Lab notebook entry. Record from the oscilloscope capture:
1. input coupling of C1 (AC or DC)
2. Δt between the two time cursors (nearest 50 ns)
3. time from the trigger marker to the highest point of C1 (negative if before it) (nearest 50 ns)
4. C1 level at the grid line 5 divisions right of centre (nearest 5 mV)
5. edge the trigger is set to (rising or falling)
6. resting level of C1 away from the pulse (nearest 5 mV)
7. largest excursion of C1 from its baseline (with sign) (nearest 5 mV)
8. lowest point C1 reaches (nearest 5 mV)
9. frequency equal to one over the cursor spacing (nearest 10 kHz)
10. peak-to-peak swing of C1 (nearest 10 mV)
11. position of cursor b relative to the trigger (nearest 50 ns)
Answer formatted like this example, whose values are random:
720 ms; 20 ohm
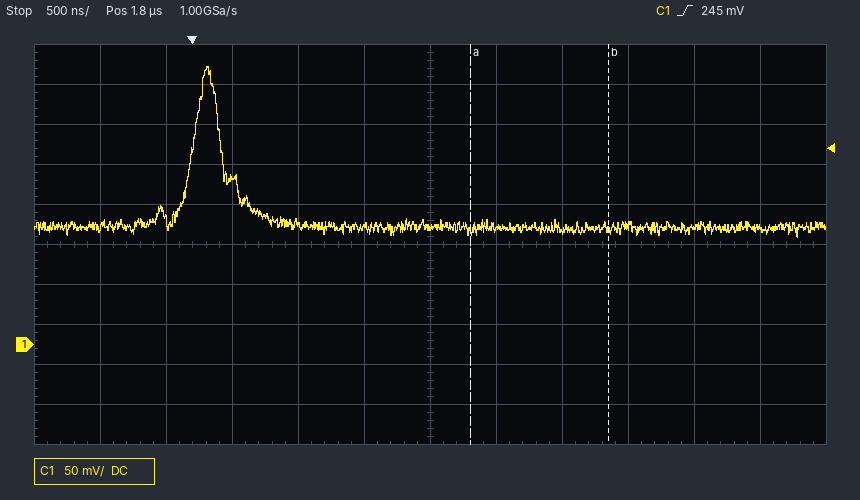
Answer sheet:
DC; 1.05 µs; +100 ns; 145 mV; rising; 145 mV; +200 mV; 135 mV; 950 kHz; 210 mV; +3.15 µs
